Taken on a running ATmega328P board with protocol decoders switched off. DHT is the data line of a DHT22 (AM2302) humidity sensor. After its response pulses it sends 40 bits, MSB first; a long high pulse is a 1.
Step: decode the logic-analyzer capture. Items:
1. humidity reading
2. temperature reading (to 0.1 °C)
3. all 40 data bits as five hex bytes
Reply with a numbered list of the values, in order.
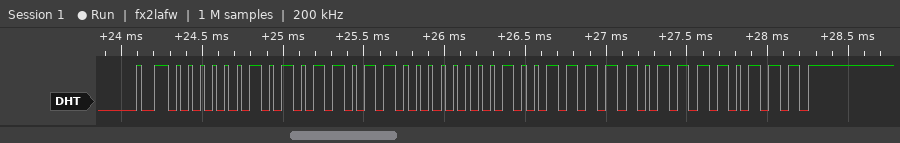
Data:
1. 69.4 %
2. 31.8 °C
3. 02 B6 01 3E F7
